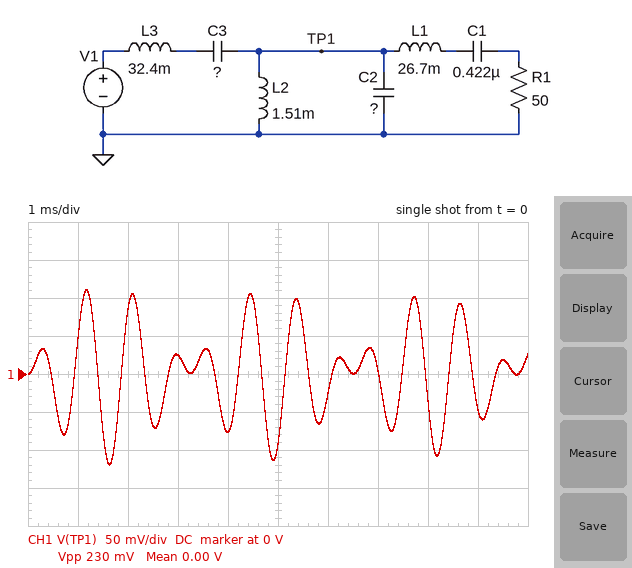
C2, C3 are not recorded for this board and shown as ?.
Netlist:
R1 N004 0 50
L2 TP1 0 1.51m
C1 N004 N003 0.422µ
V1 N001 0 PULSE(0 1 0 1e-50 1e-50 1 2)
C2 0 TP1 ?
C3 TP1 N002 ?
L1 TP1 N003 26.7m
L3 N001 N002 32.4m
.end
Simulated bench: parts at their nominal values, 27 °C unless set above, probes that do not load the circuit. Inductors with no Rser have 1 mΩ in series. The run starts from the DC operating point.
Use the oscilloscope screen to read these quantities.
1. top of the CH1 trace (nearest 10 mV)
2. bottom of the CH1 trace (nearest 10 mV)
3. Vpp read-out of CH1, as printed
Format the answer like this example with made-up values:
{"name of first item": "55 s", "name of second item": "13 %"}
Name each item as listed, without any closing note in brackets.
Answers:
{"top of the CH1 trace": "110 mV", "bottom of the CH1 trace": "-120 mV", "Vpp read-out of CH1, as printed": "230 mV"}
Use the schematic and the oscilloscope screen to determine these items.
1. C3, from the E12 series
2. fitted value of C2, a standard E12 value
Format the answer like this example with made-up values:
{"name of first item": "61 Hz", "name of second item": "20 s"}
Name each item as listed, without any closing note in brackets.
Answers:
{"C3, from the E12 series": "560 nF", "fitted value of C2, a standard E12 value": "18 µF"}
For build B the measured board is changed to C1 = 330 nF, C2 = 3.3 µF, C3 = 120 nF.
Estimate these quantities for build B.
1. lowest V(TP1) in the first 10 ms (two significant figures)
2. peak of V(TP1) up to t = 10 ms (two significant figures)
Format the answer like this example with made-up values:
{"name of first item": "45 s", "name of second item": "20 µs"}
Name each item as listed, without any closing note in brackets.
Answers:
{"lowest V(TP1) in the first 10 ms": "-150 mV", "peak of V(TP1) up to t = 10 ms": "160 mV"}
